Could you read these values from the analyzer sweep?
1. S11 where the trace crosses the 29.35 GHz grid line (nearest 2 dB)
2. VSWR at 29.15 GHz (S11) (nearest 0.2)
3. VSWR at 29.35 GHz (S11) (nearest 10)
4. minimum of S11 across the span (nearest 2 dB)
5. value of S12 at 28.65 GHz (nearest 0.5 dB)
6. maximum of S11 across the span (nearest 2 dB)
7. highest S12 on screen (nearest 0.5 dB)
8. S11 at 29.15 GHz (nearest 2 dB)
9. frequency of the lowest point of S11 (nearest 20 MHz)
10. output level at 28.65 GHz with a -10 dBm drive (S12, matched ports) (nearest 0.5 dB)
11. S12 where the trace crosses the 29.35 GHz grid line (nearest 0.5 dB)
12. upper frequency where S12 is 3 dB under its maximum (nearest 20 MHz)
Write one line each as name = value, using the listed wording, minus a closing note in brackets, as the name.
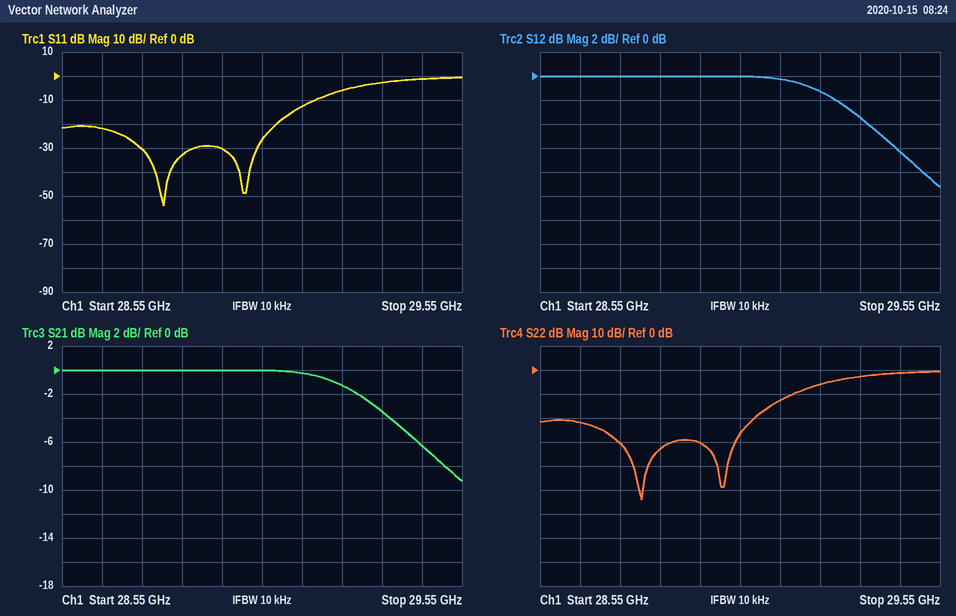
S11 where the trace crosses the 29.35 GHz grid line = -2 dB
VSWR at 29.15 GHz (S11) = 1.6
VSWR at 29.35 GHz (S11) = 10
minimum of S11 across the span = -54 dB
value of S12 at 28.65 GHz = 0.0 dB
maximum of S11 across the span = 0 dB
highest S12 on screen = 0.0 dB
S11 at 29.15 GHz = -12 dB
frequency of the lowest point of S11 = 28.80 GHz
output level at 28.65 GHz with a -10 dBm drive (S12, matched ports) = -10.0 dBm
S12 where the trace crosses the 29.35 GHz grid line = -3.5 dB
upper frequency where S12 is 3 dB under its maximum = 29.34 GHz
